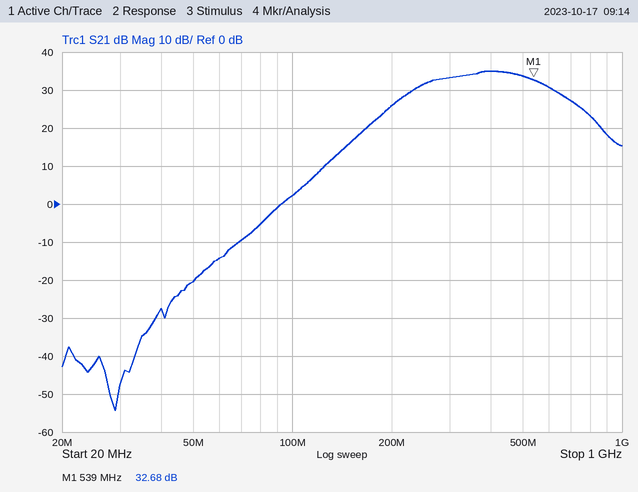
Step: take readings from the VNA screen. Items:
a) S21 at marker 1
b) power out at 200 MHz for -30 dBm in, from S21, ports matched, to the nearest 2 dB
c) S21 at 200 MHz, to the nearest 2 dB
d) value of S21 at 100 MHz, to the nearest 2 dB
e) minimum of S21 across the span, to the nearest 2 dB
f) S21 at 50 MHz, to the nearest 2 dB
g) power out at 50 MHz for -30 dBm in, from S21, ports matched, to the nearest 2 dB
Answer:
32.68 dB
-4 dBm
26 dB
2 dB
-54 dB
-20 dB
-50 dBm
